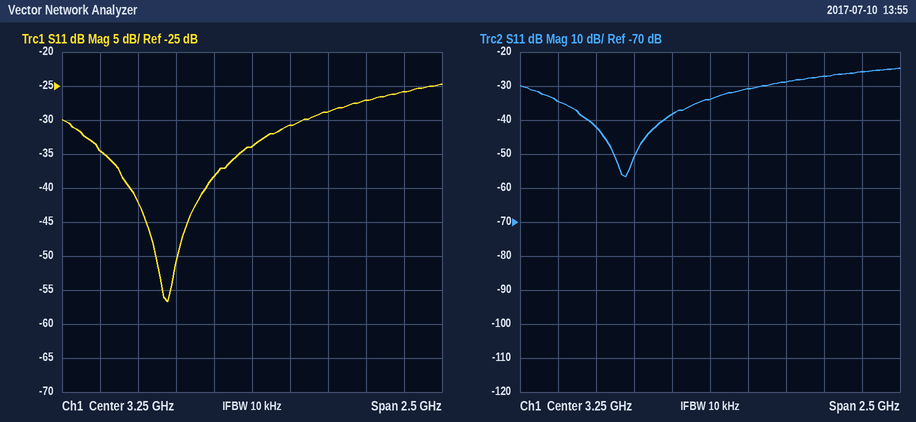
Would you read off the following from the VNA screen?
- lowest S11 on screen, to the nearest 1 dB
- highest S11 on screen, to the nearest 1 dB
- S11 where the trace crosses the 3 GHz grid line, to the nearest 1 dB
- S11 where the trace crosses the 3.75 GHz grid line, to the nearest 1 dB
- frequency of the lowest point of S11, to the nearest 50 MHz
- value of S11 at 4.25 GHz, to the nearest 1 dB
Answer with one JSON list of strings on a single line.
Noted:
["-57 dB", "-25 dB", "-38 dB", "-29 dB", "2.70 GHz", "-26 dB"]
